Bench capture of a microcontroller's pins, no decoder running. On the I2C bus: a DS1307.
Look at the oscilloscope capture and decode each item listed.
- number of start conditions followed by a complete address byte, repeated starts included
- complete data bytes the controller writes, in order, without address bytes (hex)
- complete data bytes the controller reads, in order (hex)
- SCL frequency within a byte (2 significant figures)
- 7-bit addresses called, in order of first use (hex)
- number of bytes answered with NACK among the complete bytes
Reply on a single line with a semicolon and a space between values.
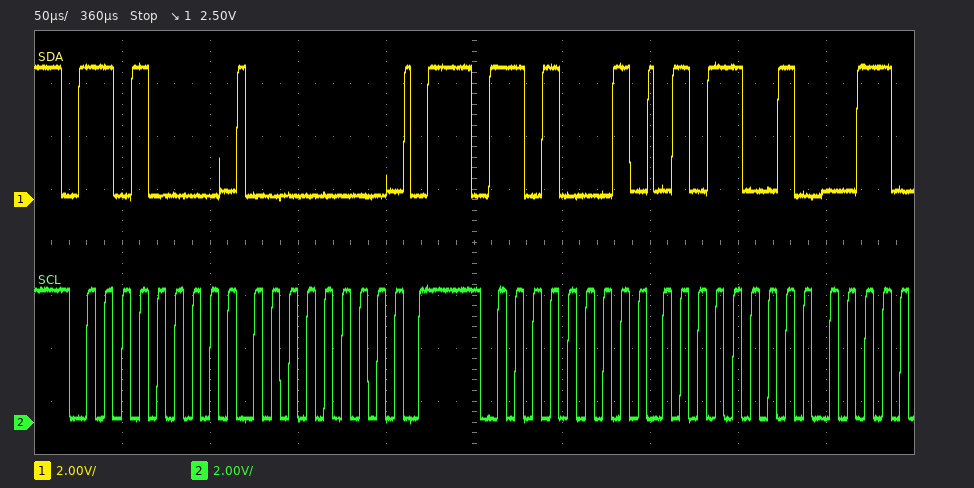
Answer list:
2; 00; 59; 100 kHz; 0x68; 0
